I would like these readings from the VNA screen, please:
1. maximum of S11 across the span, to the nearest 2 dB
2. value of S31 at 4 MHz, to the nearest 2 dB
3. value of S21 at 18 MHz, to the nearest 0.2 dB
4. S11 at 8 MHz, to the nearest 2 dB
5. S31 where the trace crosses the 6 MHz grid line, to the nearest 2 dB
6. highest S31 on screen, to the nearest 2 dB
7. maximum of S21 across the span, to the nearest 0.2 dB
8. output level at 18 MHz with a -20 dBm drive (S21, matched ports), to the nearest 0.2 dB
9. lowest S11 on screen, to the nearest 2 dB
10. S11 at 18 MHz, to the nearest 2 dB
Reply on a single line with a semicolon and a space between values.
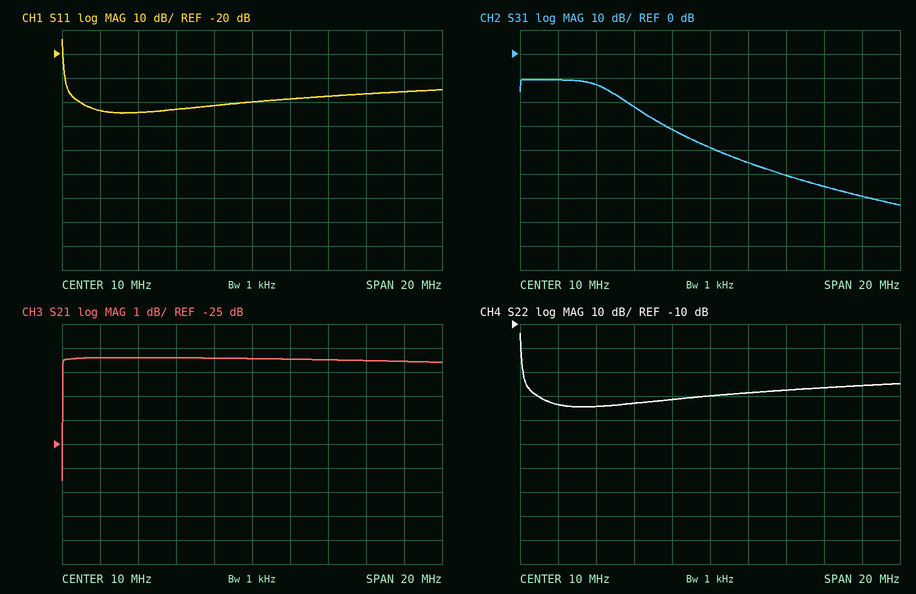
-14 dB; -12 dB; -21.6 dB; -42 dB; -22 dB; -10 dB; -21.4 dB; -41.6 dBm; -44 dB; -36 dB
